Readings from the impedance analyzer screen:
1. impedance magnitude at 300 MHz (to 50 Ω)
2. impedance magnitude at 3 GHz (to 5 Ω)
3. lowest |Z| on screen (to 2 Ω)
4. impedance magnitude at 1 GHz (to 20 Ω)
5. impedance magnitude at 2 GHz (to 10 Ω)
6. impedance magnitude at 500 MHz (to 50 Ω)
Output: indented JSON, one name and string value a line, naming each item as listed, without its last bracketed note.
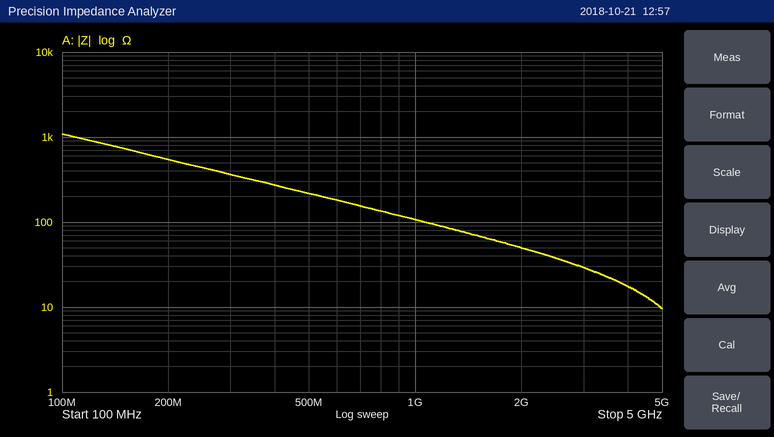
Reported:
{
  "impedance magnitude at 300 MHz": "350 Ω",
  "impedance magnitude at 3 GHz": "30 Ω",
  "lowest |Z| on screen": "10 Ω",
  "impedance magnitude at 1 GHz": "100 Ω",
  "impedance magnitude at 2 GHz": "50 Ω",
  "impedance magnitude at 500 MHz": "200 Ω"
}
